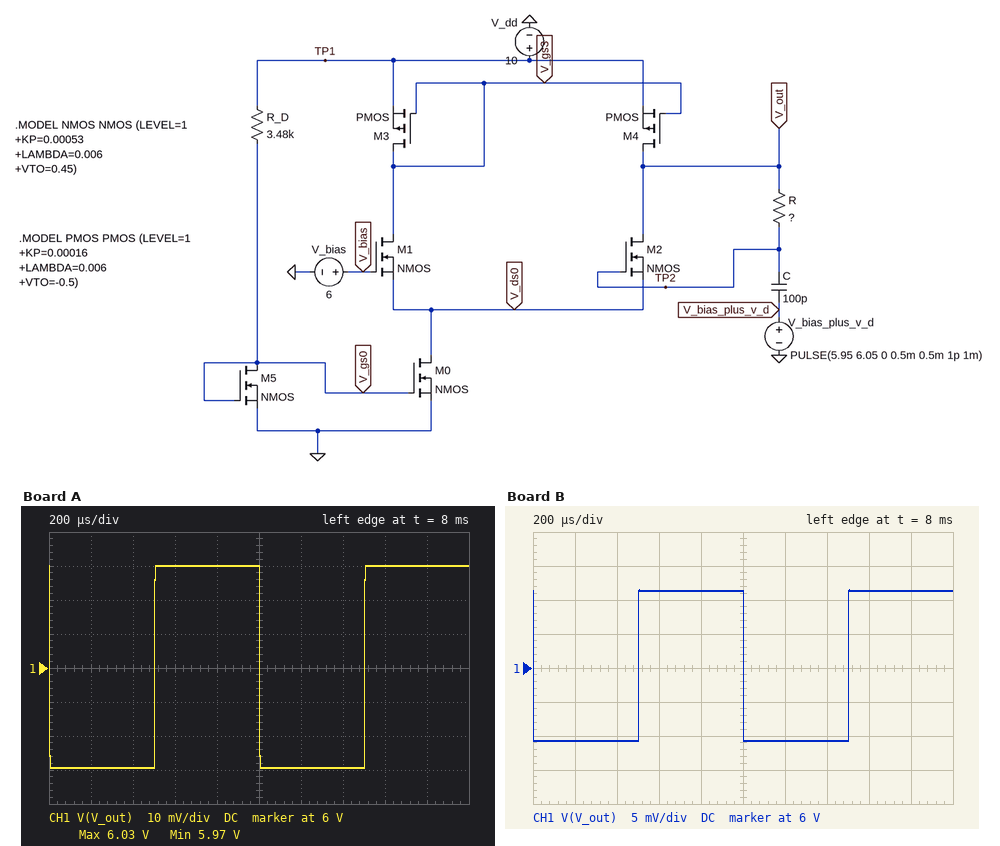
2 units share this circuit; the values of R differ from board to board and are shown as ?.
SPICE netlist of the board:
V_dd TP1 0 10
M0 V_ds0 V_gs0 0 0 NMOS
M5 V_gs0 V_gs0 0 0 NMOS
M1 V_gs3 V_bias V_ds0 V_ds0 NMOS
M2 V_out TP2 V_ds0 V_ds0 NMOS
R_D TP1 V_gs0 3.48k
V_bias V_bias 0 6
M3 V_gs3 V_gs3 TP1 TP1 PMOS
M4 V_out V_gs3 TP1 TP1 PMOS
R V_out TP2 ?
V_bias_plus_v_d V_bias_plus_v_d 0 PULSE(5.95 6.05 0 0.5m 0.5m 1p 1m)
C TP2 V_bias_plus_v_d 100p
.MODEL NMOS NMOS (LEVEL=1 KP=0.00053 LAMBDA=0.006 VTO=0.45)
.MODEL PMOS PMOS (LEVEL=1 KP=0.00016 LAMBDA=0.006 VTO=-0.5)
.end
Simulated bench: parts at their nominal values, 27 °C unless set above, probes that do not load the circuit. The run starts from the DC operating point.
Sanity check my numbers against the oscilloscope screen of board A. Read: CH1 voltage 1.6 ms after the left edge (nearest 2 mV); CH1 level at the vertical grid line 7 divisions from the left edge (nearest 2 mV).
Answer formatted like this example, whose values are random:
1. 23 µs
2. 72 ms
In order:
1. 6.030 V
2. 5.970 V
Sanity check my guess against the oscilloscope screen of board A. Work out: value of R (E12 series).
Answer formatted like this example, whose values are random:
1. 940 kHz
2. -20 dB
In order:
1. 1.5 MΩ
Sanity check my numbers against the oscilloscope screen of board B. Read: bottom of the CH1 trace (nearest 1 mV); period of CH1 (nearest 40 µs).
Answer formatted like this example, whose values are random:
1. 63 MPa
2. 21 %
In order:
1. 5.989 V
2. 1.00 ms
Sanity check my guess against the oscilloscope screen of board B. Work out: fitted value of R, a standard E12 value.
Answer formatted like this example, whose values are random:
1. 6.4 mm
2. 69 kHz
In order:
1. 560 kΩ
